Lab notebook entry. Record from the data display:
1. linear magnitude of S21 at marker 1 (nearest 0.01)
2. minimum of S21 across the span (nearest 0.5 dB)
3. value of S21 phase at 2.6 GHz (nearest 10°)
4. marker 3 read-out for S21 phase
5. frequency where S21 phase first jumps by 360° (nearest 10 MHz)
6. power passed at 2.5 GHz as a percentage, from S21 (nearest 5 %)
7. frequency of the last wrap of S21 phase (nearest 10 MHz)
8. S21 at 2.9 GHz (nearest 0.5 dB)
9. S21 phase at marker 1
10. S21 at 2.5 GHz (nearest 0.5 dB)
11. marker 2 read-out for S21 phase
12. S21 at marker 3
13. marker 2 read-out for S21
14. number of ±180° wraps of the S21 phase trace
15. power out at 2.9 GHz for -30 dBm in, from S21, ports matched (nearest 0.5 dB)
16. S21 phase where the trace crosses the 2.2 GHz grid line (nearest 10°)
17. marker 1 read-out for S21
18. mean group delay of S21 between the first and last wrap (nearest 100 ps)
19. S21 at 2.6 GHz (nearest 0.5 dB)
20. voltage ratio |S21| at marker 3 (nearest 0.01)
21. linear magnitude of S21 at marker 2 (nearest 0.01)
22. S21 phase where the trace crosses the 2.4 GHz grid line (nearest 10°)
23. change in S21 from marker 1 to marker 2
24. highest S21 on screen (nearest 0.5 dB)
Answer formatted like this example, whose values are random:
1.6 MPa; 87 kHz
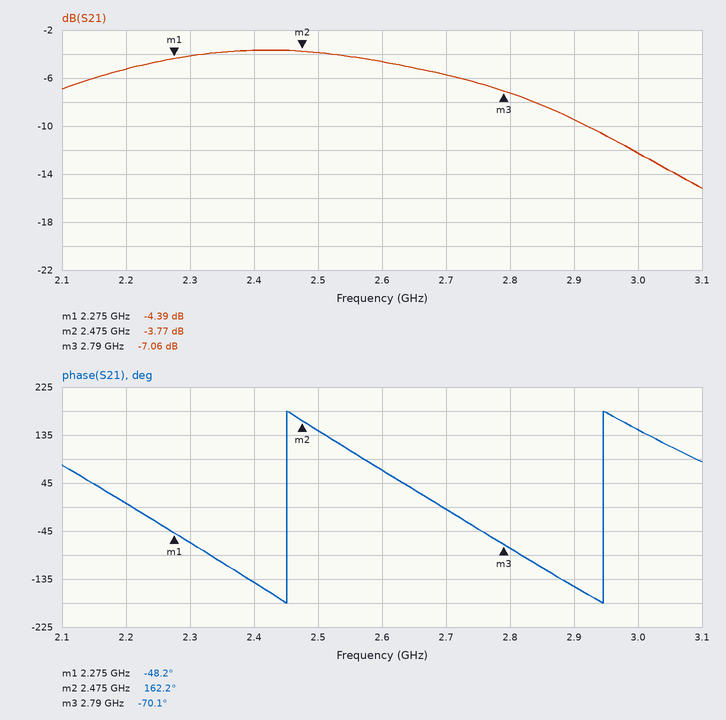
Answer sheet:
0.60; -15.0 dB; 70°; -70.1°; 2.45 GHz; 40 %; 2.95 GHz; -9.5 dB; -48.2°; -4.0 dB; 162.2°; -7.06 dB; -3.77 dB; 2; -39.5 dBm; 10°; -4.39 dB; 2.0 ns; -4.5 dB; 0.44; 0.65; -140°; 0.62 dB; -3.5 dB
